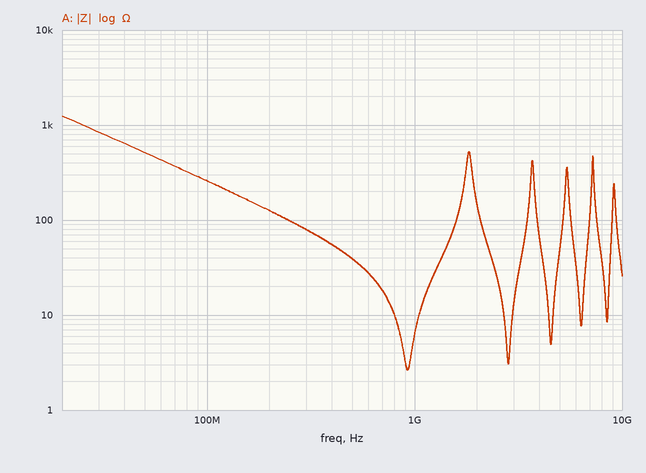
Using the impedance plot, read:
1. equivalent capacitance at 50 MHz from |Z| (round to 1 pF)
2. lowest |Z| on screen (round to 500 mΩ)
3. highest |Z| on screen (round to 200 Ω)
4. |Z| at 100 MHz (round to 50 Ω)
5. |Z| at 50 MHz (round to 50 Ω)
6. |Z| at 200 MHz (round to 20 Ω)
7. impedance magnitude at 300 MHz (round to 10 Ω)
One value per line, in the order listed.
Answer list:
6 pF
2.5 Ω
1.2 kΩ
250 Ω
500 Ω
120 Ω
80 Ω
